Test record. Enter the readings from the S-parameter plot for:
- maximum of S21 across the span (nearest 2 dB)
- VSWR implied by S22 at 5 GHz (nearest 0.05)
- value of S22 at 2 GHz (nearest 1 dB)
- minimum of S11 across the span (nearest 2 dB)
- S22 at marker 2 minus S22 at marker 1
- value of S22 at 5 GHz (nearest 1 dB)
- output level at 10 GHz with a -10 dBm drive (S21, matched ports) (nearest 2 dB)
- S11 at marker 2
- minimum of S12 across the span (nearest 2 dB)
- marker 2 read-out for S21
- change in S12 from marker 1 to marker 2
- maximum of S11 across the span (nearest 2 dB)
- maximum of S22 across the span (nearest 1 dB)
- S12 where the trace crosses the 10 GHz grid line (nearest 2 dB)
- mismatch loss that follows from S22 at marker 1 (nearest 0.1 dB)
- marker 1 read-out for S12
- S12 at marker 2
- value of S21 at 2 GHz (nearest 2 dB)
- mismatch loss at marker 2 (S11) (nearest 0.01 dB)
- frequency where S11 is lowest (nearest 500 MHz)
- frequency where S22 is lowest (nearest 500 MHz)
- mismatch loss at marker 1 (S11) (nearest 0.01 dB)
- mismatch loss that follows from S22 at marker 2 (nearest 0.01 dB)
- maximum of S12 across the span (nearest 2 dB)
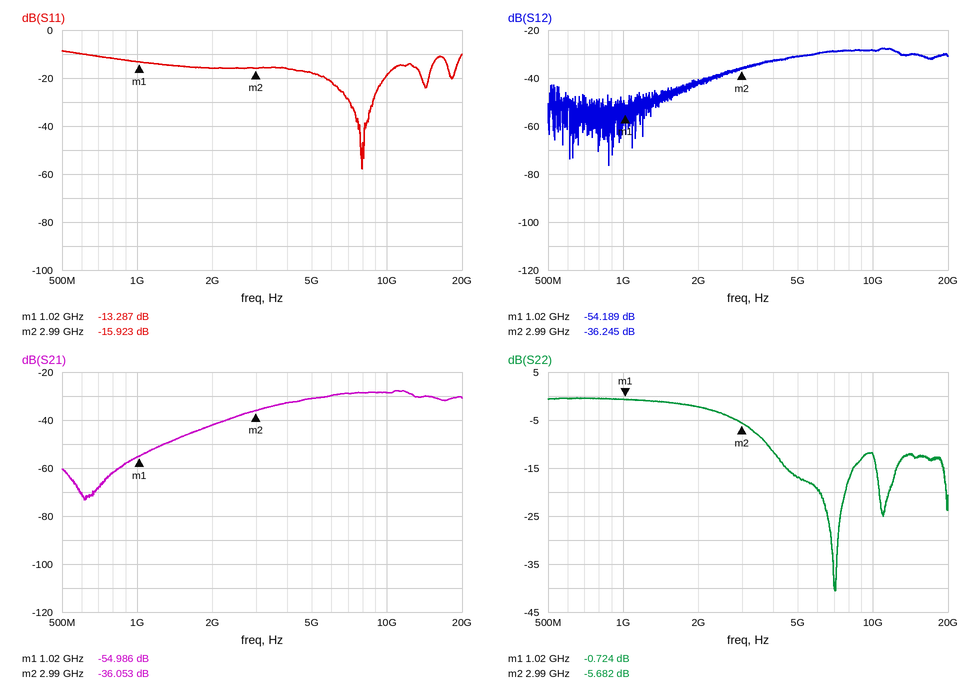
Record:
-28 dB
1.35
-2 dB
-58 dB
-4.958 dB
-17 dB
-38 dBm
-15.923 dB
-76 dB
-36.053 dB
17.944 dB
-8 dB
0 dB
-28 dB
8.1 dB
-54.189 dB
-36.245 dB
-42 dB
0.11 dB
8.0 GHz
7.0 GHz
0.21 dB
1.37 dB
-28 dB
